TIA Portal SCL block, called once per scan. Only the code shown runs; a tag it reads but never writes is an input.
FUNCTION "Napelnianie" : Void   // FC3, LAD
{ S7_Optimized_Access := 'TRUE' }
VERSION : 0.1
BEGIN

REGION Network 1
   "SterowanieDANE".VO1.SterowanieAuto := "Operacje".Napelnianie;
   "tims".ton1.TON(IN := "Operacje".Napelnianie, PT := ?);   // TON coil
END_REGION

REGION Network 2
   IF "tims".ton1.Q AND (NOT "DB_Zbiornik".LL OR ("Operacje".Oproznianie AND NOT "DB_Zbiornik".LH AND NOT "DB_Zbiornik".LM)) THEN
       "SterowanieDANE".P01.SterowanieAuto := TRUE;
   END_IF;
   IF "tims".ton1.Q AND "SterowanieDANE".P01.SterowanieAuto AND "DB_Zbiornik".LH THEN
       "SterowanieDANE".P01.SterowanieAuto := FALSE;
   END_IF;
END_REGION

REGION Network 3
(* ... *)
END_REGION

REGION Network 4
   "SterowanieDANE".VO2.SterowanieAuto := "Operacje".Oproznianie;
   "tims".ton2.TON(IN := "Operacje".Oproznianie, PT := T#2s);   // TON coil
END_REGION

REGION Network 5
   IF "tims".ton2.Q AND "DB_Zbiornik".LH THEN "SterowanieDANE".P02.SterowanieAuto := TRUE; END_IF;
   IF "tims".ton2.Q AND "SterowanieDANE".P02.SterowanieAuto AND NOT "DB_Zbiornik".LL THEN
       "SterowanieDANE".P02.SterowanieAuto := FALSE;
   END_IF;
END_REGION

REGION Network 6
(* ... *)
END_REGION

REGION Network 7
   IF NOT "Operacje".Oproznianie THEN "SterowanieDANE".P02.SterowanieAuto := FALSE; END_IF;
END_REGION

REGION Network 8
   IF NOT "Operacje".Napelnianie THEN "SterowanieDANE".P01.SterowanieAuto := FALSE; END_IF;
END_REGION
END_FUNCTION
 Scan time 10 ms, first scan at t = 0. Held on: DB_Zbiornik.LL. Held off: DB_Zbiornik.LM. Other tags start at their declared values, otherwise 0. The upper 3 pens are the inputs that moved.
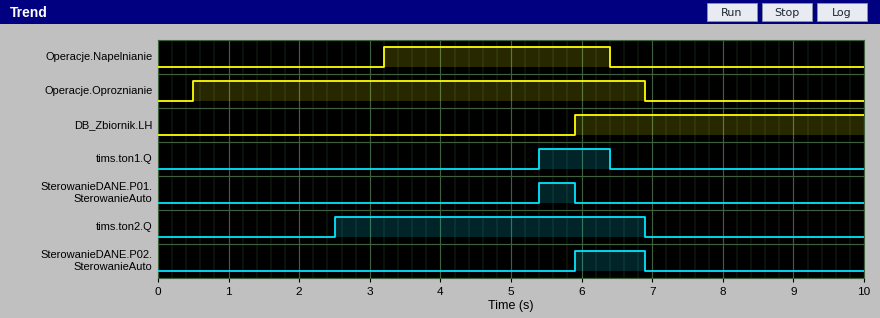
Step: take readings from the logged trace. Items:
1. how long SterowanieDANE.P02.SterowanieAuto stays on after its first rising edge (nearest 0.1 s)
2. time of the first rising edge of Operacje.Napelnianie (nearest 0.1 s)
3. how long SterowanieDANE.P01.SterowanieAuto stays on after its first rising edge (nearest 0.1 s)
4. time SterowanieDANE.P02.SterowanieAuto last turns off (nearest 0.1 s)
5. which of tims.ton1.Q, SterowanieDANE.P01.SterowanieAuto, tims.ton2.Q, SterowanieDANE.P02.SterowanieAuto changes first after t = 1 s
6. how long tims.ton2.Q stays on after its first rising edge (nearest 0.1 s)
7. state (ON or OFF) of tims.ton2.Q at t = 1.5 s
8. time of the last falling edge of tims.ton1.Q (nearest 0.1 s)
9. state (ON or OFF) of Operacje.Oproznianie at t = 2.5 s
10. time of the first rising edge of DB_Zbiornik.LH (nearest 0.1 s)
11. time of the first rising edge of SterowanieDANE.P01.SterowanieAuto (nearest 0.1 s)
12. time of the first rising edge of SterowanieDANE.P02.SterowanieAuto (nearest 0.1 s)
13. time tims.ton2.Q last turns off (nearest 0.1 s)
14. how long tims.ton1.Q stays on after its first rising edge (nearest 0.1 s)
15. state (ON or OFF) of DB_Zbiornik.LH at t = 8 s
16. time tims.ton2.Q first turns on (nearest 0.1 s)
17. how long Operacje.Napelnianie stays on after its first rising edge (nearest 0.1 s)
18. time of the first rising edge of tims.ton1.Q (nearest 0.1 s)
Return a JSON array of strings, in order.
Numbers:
["1.0 s", "3.2 s", "0.5 s", "6.9 s", "tims.ton2.Q", "4.4 s", "OFF", "6.4 s", "ON", "5.9 s", "5.4 s", "5.9 s", "6.9 s", "1.0 s", "ON", "2.5 s", "3.2 s", "5.4 s"]
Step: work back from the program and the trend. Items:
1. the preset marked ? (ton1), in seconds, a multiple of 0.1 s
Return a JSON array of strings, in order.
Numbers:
["2.2 s"]
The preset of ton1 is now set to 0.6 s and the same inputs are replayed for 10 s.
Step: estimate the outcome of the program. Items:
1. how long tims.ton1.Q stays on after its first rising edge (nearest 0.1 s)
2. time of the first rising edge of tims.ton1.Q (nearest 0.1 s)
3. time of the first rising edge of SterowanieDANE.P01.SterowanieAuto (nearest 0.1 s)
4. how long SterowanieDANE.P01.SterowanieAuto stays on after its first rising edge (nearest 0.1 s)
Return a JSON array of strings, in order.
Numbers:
["2.6 s", "3.8 s", "3.8 s", "2.1 s"]
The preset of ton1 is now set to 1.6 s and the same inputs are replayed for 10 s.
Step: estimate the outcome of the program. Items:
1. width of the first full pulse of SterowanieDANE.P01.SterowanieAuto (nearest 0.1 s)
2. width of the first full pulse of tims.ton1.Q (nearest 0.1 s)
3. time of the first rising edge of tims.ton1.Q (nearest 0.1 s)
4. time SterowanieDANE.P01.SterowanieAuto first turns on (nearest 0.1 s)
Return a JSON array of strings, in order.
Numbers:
["1.1 s", "1.6 s", "4.8 s", "4.8 s"]
